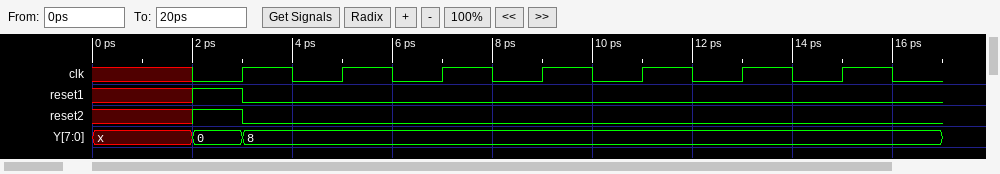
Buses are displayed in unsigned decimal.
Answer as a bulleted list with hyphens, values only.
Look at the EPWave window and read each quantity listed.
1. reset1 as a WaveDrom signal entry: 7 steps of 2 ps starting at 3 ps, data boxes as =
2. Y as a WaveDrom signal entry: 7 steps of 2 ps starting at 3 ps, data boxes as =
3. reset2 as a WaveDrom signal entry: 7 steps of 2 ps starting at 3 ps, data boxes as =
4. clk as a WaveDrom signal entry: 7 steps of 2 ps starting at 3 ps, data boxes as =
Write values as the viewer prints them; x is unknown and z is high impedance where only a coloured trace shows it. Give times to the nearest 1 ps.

- {name: 'reset1', wave: '0......'}
- {name: 'Y', wave: '=......', data: '8'}
- {name: 'reset2', wave: '0......'}
- {name: 'clk', wave: 'p......'}
